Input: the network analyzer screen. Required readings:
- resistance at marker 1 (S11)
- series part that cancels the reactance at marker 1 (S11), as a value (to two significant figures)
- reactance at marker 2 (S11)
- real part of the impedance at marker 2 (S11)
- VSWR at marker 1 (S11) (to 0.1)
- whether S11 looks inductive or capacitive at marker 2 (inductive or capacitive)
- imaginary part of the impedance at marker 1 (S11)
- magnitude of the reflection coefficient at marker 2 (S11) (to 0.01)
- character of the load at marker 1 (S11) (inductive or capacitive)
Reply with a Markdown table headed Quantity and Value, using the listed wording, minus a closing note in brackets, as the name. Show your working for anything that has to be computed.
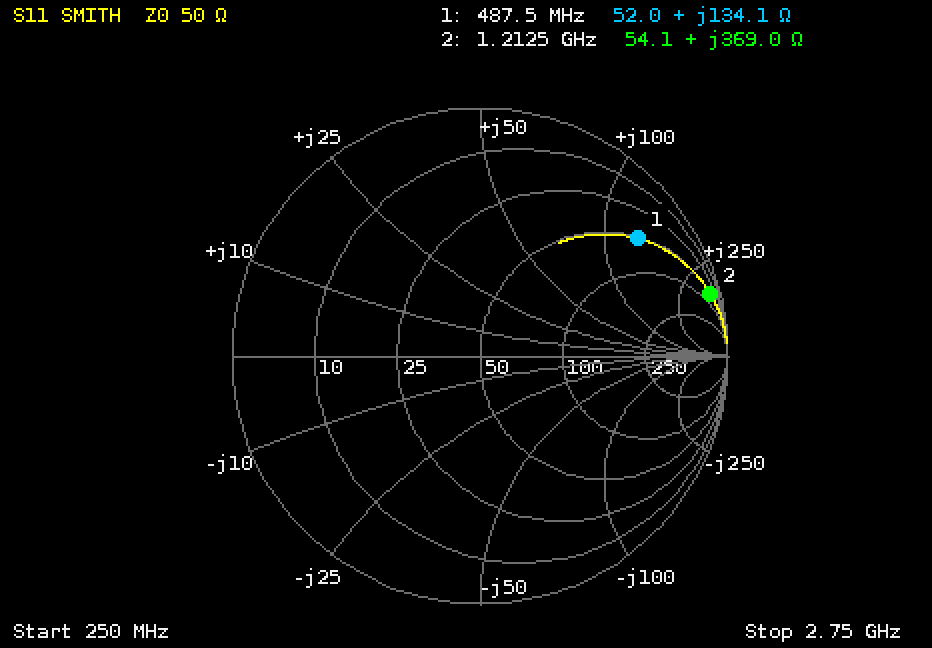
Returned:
| Quantity | Value |
|---|---|
| resistance at marker 1 | 52.0 Ω |
| series part that cancels the reactance at marker 1 (S11), as a value | C = 1/(2π × 487.5 MHz × 134.1 Ω) ≈ 2.4 pF |
| reactance at marker 2 | +369.0 Ω |
| real part of the impedance at marker 2 | 54.1 Ω |
| VSWR at marker 1 (S11) | 8.8 |
| whether S11 looks inductive or capacitive at marker 2 | inductive |
| imaginary part of the impedance at marker 1 | +134.1 Ω |
| magnitude of the reflection coefficient at marker 2 (S11) | 0.96 |
| character of the load at marker 1 (S11) | inductive |
